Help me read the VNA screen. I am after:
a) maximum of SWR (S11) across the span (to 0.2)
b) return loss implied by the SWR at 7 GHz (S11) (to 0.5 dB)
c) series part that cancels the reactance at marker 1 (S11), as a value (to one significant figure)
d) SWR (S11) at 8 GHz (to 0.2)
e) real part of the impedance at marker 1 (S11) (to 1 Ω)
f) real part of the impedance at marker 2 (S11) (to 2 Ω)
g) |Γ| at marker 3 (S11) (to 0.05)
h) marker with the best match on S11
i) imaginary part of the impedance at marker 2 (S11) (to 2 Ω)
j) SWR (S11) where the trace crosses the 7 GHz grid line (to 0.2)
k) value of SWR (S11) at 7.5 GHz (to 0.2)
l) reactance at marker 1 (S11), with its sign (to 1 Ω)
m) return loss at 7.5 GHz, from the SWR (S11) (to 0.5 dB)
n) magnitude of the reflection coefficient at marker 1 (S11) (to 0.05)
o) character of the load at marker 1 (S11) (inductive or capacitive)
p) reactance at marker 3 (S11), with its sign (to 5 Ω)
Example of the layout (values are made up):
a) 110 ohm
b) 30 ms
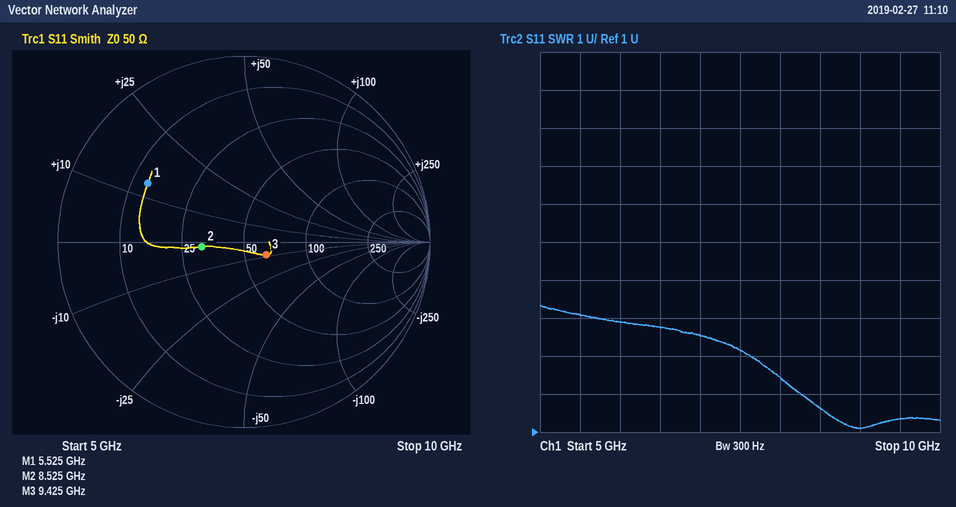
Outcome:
a) 4.4
b) 5.0 dB
c) 2 pF
d) 2.4
e) 13 Ω
f) 32 Ω
g) 0.15
h) marker 3
i) -2 Ω
j) 3.6
k) 3.2
l) +13 Ω
m) 5.5 dB
n) 0.60
o) inductive
p) -10 Ω
